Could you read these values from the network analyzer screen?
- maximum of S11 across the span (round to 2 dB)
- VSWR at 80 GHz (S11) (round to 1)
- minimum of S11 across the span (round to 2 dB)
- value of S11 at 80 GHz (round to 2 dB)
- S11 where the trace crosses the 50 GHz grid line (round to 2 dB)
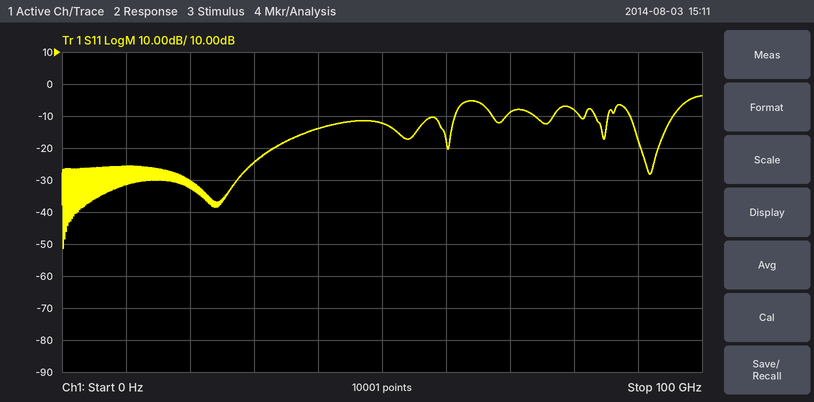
-4 dB
2
-52 dB
-8 dB
-12 dB
